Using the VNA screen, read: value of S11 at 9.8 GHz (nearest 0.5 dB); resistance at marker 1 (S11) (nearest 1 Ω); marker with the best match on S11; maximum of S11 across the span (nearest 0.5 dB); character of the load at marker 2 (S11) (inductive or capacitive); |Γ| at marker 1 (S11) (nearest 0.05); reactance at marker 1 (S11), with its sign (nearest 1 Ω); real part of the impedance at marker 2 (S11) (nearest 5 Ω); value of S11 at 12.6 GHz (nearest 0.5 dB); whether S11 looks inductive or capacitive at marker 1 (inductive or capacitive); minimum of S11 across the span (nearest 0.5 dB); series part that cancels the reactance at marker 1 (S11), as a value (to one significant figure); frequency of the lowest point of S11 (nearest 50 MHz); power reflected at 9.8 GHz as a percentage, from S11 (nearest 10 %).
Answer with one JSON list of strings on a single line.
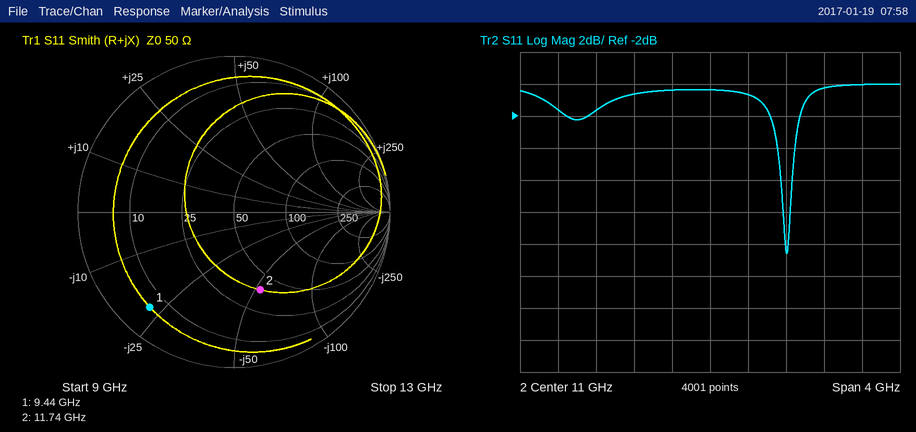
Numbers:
["-1.5 dB", "6 Ω", "marker 2", "0.0 dB", "capacitive", "0.80", "-22 Ω", "40 Ω", "0.0 dB", "capacitive", "-10.5 dB", "400 pH", "11.80 GHz", "70 %"]
